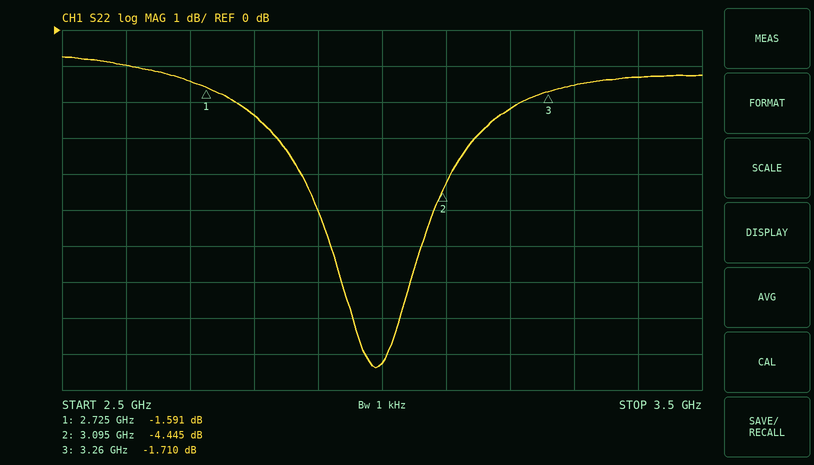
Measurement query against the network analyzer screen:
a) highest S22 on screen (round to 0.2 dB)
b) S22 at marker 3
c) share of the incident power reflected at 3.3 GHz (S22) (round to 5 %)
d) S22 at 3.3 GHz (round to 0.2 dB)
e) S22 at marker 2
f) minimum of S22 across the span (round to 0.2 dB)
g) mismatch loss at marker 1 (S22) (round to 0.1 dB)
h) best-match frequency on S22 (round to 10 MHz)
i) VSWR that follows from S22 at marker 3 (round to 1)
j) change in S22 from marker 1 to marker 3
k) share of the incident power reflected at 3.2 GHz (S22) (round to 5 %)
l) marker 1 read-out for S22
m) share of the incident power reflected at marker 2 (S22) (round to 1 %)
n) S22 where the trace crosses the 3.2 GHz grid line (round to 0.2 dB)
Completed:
-0.8 dB
-1.710 dB
70 %
-1.6 dB
-4.445 dB
-9.4 dB
5.1 dB
2.99 GHz
10
-0.119 dB
60 %
-1.591 dB
36 %
-2.2 dB
